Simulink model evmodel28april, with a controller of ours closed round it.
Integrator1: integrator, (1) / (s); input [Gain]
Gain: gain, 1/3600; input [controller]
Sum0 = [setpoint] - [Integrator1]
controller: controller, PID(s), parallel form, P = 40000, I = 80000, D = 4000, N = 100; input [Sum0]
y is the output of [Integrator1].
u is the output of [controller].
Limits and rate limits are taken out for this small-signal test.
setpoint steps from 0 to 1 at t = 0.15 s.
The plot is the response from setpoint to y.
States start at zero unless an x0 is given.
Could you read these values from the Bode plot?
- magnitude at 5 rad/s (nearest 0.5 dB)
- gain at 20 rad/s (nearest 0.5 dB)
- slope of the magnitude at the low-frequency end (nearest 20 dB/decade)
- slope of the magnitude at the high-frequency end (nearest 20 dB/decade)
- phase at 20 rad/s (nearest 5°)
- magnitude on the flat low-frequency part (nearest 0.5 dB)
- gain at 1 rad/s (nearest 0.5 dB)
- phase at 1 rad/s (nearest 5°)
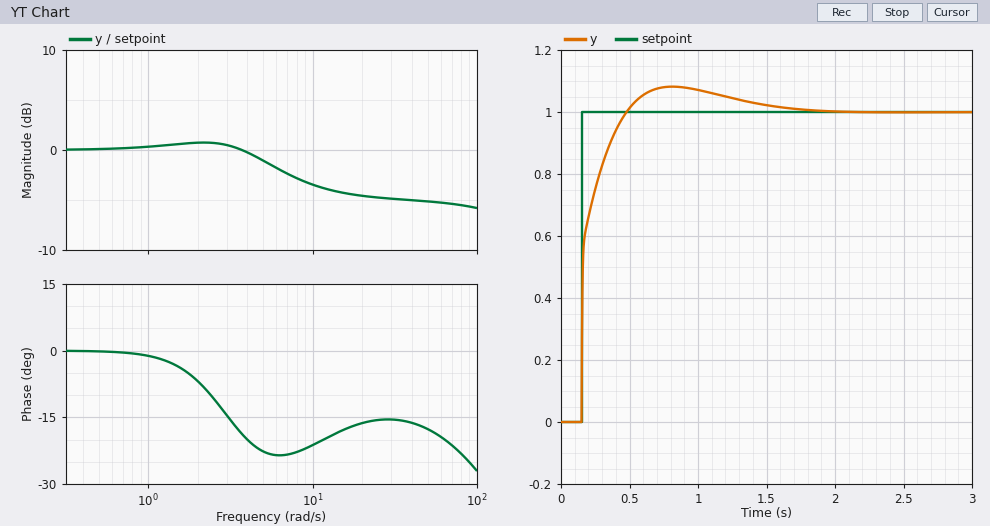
-1.0 dB
-4.5 dB
0 dB/decade
0 dB/decade
-15°
0.0 dB
0.5 dB
0°
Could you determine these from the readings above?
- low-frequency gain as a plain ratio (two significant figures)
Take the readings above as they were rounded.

1.0
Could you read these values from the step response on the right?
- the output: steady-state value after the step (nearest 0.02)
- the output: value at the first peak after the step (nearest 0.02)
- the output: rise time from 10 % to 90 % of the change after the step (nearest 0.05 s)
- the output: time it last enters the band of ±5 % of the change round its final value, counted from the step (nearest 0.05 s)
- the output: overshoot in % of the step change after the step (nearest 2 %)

1.00
1.08
0.20 s
1.05 s
8 %
